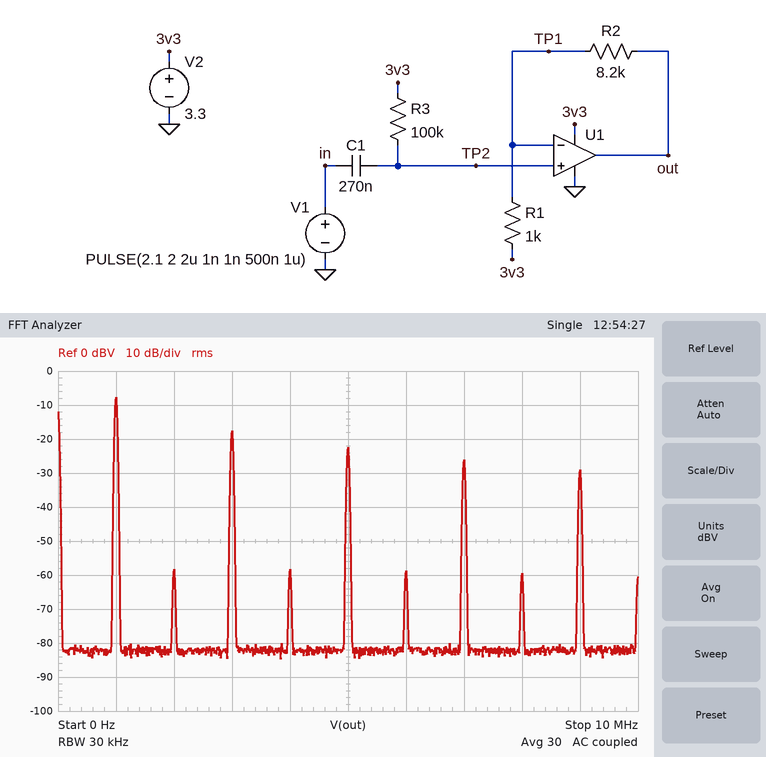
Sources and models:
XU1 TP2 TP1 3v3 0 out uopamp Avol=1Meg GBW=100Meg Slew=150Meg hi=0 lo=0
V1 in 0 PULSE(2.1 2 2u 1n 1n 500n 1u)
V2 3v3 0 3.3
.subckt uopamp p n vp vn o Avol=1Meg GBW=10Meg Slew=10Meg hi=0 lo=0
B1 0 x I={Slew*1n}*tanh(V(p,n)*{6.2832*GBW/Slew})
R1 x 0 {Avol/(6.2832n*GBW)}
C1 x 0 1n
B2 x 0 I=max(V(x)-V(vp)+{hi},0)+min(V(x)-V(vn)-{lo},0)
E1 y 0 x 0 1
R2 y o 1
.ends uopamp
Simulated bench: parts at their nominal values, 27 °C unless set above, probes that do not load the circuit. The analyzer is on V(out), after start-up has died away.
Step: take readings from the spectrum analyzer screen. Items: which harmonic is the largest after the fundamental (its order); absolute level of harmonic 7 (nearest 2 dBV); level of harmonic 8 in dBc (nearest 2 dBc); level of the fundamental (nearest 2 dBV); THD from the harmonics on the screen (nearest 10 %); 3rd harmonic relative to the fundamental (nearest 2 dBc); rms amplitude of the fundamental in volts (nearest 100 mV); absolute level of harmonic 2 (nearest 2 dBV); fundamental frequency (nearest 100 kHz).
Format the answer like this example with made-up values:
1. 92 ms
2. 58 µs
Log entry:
1. 3
2. -26 dBV
3. -52 dBc
4. -8 dBV
5. 40 %
6. -10 dBc
7. 400 mV
8. -58 dBV
9. 1.0 MHz
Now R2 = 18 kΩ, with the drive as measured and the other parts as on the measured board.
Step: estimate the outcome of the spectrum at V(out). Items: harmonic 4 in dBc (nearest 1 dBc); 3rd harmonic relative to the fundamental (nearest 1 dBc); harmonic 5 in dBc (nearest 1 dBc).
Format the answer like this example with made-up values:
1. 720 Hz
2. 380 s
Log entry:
1. -52 dBc
2. -11 dBc
3. -17 dBc
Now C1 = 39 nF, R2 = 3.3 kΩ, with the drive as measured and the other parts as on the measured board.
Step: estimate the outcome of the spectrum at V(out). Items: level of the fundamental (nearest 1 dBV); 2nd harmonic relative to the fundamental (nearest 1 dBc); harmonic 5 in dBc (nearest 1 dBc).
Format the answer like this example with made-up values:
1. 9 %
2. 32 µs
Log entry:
1. -14 dBV
2. -52 dBc
3. -14 dBc
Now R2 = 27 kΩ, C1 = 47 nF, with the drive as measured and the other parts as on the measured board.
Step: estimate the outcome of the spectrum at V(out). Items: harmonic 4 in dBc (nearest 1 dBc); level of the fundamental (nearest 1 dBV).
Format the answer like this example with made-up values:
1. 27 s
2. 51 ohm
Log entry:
1. -53 dBc
2. 2 dBV
